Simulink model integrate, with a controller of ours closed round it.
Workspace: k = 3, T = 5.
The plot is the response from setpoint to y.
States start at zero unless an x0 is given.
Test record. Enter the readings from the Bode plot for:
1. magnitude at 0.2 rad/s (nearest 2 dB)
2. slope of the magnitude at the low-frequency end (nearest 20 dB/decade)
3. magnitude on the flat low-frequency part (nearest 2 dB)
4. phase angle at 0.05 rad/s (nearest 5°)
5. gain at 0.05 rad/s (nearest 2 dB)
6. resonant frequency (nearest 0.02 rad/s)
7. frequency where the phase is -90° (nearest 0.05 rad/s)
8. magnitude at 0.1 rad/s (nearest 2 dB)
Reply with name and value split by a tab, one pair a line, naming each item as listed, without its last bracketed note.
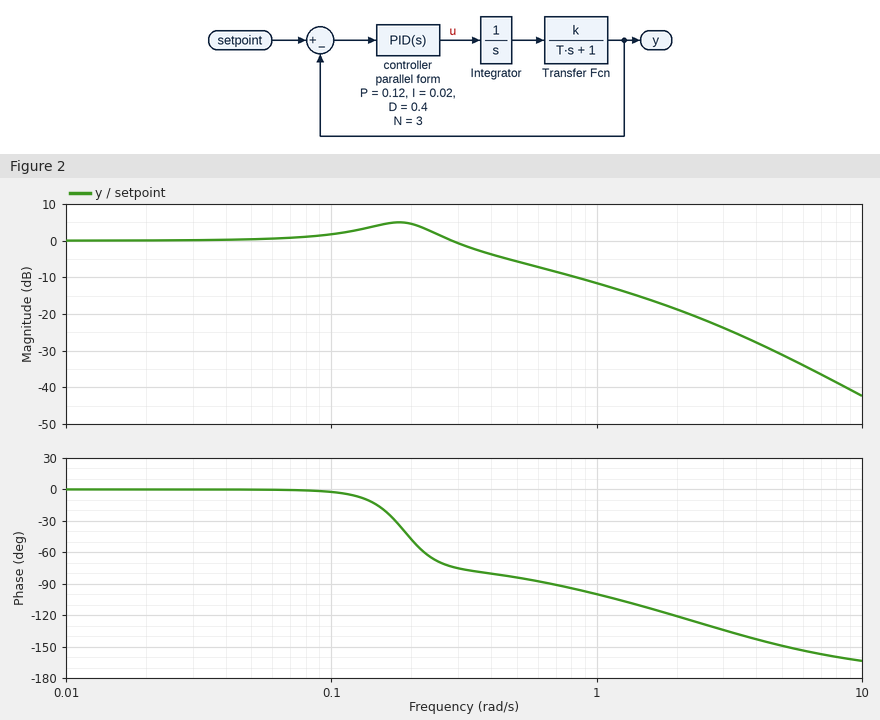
magnitude at 0.2 rad/s	4 dB
slope of the magnitude at the low-frequency end	0 dB/decade
magnitude on the flat low-frequency part	0 dB
phase angle at 0.05 rad/s	0°
gain at 0.05 rad/s	0 dB
resonant frequency	0.18 rad/s
frequency where the phase is -90°	0.65 rad/s
magnitude at 0.1 rad/s	2 dB
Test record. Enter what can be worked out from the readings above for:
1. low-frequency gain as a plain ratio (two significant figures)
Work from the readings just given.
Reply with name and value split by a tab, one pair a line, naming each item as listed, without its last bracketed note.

low-frequency gain as a plain ratio	1.0
